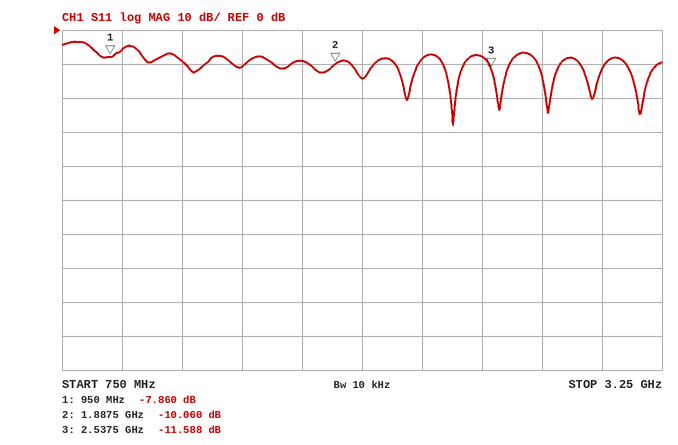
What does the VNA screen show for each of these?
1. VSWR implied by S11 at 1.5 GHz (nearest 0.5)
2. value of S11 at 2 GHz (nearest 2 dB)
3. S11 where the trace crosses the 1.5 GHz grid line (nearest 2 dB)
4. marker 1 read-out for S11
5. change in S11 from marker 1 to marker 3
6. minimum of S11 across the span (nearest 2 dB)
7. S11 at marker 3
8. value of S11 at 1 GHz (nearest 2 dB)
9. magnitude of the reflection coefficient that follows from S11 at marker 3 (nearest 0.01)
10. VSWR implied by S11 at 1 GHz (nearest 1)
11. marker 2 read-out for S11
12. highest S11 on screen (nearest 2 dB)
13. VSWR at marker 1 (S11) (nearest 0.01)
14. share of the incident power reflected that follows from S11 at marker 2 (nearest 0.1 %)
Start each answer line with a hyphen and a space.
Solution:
- 2.0
- -14 dB
- -10 dB
- -7.860 dB
- -3.728 dB
- -28 dB
- -11.588 dB
- -6 dB
- 0.26
- 3
- -10.060 dB
- -4 dB
- 2.36
- 9.9 %
